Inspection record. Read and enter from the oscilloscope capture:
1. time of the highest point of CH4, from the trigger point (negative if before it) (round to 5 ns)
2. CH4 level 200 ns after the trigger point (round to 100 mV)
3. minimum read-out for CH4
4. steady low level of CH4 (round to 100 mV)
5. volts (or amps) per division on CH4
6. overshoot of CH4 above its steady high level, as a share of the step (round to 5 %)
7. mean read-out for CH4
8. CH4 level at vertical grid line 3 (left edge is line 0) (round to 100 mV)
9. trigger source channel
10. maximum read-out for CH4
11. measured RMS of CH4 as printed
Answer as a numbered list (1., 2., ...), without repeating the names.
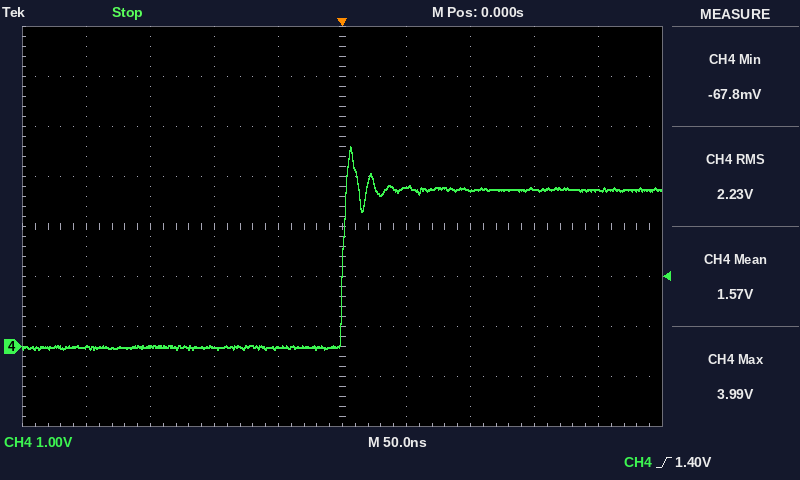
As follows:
1. +5 ns
2. 3.1 V
3. -67.8 mV
4. 0.0 V
5. 1 V
6. 25 %
7. 1.57 V
8. 0.0 V
9. CH4
10. 3.99 V
11. 2.23 V
